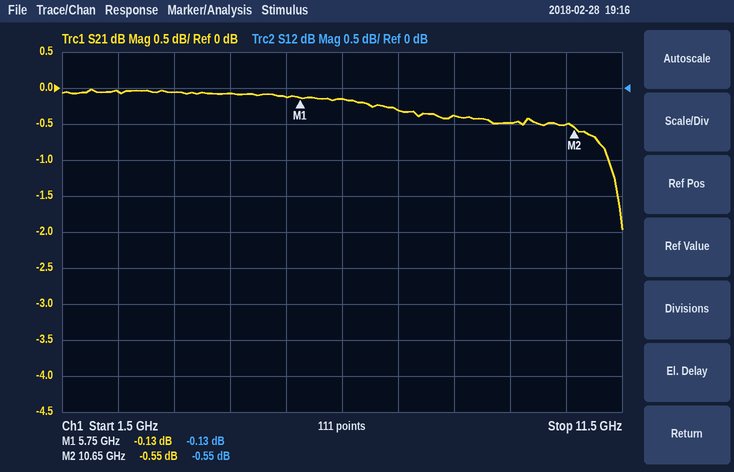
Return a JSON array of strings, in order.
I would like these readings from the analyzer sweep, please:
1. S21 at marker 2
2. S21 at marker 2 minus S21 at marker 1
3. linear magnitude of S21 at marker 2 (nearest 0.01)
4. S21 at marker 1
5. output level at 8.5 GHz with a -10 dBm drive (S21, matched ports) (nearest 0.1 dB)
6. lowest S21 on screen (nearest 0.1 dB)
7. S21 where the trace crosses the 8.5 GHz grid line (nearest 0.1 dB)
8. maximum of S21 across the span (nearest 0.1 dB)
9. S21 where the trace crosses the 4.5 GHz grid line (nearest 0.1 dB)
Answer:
["-0.55 dB", "-0.42 dB", "0.94", "-0.13 dB", "-10.4 dBm", "-2.0 dB", "-0.4 dB", "0.0 dB", "-0.1 dB"]
